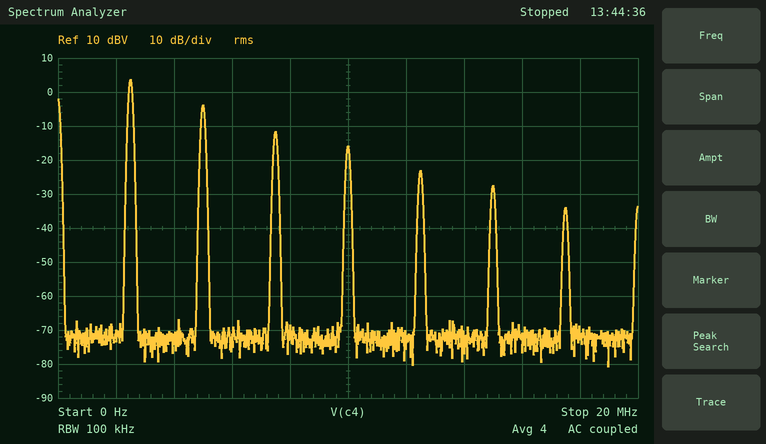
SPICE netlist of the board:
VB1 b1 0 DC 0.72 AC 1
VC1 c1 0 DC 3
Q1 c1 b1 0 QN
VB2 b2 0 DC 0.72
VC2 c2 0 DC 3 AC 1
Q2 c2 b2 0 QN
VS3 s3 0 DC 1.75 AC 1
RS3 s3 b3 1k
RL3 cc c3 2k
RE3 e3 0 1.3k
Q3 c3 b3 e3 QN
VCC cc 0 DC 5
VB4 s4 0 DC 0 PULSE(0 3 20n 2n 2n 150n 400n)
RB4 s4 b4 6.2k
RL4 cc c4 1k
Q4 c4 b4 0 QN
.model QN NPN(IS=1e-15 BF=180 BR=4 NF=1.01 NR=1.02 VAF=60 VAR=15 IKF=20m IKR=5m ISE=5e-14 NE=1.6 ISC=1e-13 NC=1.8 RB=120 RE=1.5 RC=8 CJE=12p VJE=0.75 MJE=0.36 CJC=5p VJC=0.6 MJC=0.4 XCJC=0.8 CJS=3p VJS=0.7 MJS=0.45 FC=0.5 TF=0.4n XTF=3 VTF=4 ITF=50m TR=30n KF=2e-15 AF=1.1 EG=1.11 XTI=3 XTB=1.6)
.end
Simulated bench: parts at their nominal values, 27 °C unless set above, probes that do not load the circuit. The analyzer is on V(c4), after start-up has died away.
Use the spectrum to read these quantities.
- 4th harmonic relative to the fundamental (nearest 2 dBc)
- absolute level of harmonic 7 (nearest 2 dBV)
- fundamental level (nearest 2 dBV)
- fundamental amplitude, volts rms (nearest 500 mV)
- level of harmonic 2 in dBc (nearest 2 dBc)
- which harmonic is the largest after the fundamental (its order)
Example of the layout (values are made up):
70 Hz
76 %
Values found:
-20 dBc
-34 dBV
4 dBV
1.5 V
-8 dBc
2
